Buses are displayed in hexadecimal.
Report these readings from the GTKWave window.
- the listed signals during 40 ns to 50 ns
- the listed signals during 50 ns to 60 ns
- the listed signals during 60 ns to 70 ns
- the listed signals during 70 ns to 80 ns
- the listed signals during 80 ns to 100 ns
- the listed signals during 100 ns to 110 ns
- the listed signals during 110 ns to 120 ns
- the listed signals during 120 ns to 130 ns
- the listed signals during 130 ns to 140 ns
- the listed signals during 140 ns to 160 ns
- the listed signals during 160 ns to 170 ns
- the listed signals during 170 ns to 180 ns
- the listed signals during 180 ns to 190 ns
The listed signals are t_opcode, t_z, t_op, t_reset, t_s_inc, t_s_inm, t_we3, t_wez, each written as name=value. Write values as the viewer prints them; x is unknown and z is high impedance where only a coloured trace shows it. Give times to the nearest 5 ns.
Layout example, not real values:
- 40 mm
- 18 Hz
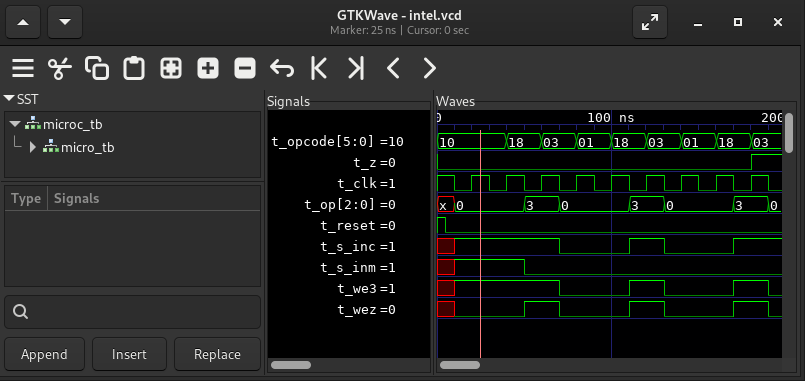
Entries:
- t_opcode=18, t_z=0, t_op=0, t_reset=0, t_s_inc=1, t_s_inm=1, t_we3=1, t_wez=0
- t_opcode=18, t_z=0, t_op=3, t_reset=0, t_s_inc=1, t_s_inm=0, t_we3=1, t_wez=1
- t_opcode=03, t_z=0, t_op=3, t_reset=0, t_s_inc=1, t_s_inm=0, t_we3=1, t_wez=1
- t_opcode=03, t_z=0, t_op=0, t_reset=0, t_s_inc=0, t_s_inm=0, t_we3=0, t_wez=0
- t_opcode=01, t_z=0, t_op=0, t_reset=0, t_s_inc=0, t_s_inm=0, t_we3=0, t_wez=0
- t_opcode=18, t_z=0, t_op=0, t_reset=0, t_s_inc=0, t_s_inm=0, t_we3=0, t_wez=0
- t_opcode=18, t_z=0, t_op=3, t_reset=0, t_s_inc=1, t_s_inm=0, t_we3=1, t_wez=1
- t_opcode=03, t_z=0, t_op=3, t_reset=0, t_s_inc=1, t_s_inm=0, t_we3=1, t_wez=1
- t_opcode=03, t_z=0, t_op=0, t_reset=0, t_s_inc=0, t_s_inm=0, t_we3=0, t_wez=0
- t_opcode=01, t_z=0, t_op=0, t_reset=0, t_s_inc=0, t_s_inm=0, t_we3=0, t_wez=0
- t_opcode=18, t_z=0, t_op=0, t_reset=0, t_s_inc=0, t_s_inm=0, t_we3=0, t_wez=0
- t_opcode=18, t_z=0, t_op=3, t_reset=0, t_s_inc=1, t_s_inm=0, t_we3=1, t_wez=1
- t_opcode=03, t_z=1, t_op=3, t_reset=0, t_s_inc=1, t_s_inm=0, t_we3=1, t_wez=1
